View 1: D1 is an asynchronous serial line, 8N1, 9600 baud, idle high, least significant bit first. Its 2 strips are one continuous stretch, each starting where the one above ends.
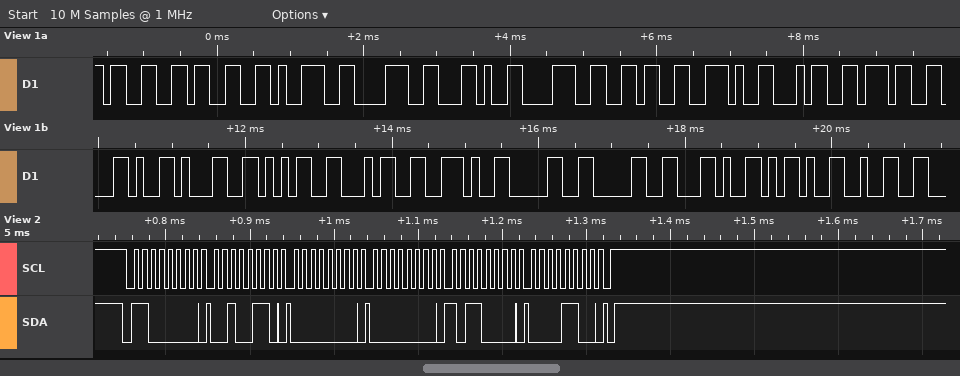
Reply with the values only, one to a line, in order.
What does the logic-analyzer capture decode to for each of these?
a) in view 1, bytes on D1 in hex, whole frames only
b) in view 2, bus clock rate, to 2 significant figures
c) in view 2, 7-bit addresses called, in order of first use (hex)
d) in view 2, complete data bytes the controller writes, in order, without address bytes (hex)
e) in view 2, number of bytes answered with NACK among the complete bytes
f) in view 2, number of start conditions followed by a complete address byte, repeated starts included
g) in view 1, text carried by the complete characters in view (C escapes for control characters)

33 33 39 38 2C 38 36 2E 34 37 2C 31 35 34 2E 30 30 2C 2D 32
100 kHz
0x60
26 00 00 B0 0C
0
1
"3398,86.47,154.00,-2"
